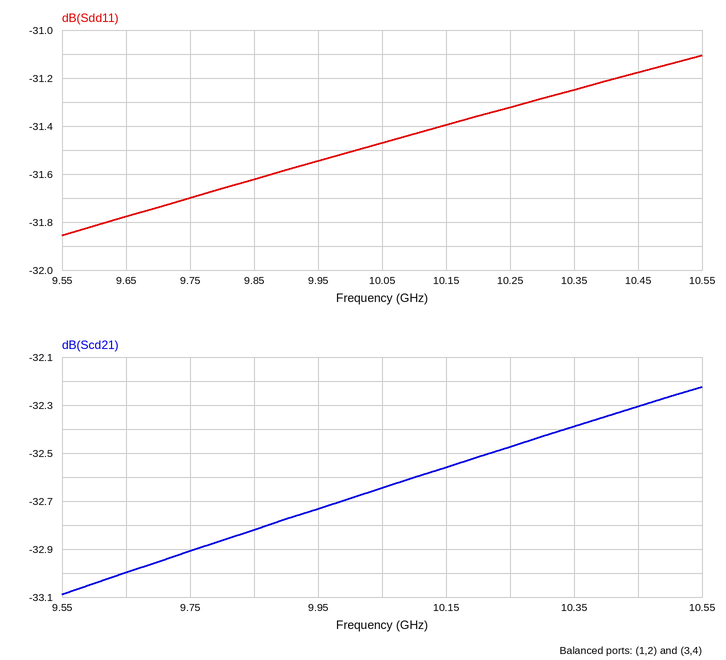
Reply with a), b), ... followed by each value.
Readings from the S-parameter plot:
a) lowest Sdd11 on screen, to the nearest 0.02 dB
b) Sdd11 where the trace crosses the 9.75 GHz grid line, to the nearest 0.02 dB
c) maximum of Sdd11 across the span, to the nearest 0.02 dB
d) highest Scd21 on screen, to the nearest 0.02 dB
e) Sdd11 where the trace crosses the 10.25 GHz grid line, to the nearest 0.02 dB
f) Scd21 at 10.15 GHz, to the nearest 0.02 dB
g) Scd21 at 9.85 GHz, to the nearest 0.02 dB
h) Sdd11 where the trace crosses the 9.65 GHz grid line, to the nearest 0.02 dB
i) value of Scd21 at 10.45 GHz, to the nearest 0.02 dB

a) -31.86 dB
b) -31.70 dB
c) -31.10 dB
d) -32.22 dB
e) -31.32 dB
f) -32.56 dB
g) -32.82 dB
h) -31.78 dB
i) -32.30 dB
